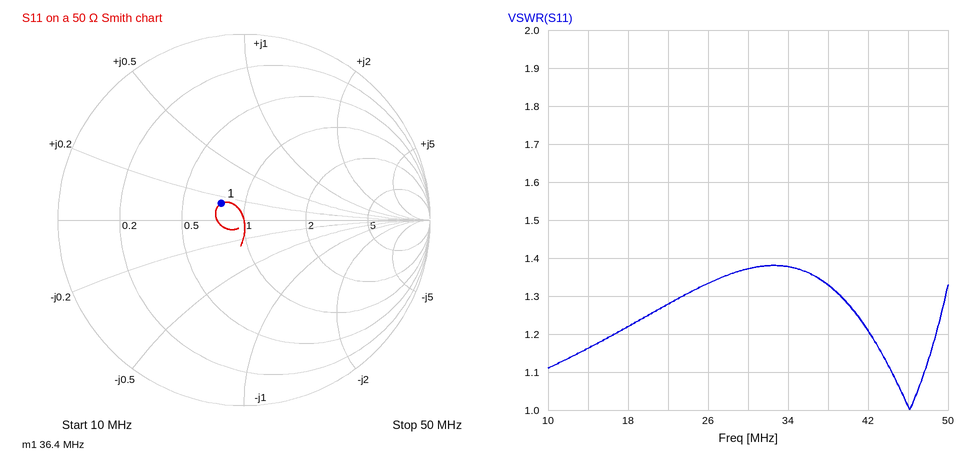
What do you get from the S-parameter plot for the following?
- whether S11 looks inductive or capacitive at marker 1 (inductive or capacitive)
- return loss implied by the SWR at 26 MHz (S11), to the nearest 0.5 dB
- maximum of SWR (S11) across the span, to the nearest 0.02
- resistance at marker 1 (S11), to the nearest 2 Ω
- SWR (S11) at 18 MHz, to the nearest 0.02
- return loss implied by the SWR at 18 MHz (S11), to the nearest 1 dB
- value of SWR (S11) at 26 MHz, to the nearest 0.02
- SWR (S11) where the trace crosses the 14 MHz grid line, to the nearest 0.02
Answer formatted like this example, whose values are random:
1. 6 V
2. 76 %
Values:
1. inductive
2. 17.0 dB
3. 1.38
4. 38 Ω
5. 1.22
6. 20 dB
7. 1.34
8. 1.16
